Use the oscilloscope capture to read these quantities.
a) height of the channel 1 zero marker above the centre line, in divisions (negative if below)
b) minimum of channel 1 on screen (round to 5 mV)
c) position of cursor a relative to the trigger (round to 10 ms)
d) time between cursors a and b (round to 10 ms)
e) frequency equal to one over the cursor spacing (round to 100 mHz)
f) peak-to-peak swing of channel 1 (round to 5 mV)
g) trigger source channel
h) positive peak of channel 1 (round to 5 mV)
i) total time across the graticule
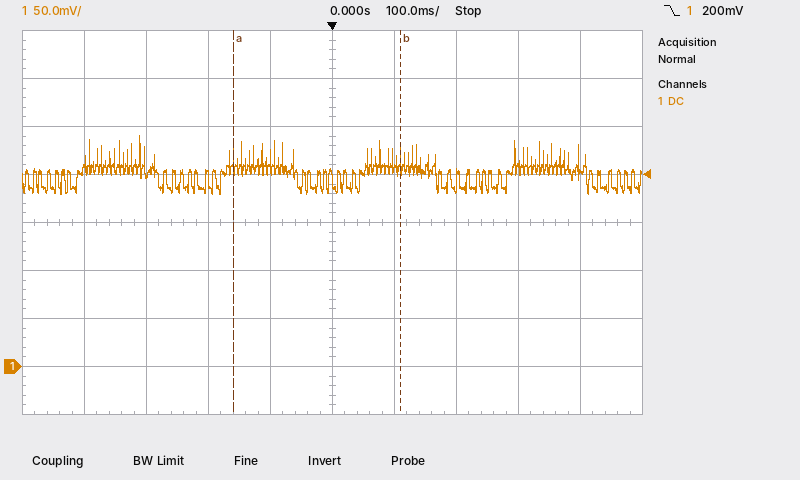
-3.0 div
180 mV
-160 ms
270 ms
3.7 Hz
60 mV
channel 1
240 mV
1 s
